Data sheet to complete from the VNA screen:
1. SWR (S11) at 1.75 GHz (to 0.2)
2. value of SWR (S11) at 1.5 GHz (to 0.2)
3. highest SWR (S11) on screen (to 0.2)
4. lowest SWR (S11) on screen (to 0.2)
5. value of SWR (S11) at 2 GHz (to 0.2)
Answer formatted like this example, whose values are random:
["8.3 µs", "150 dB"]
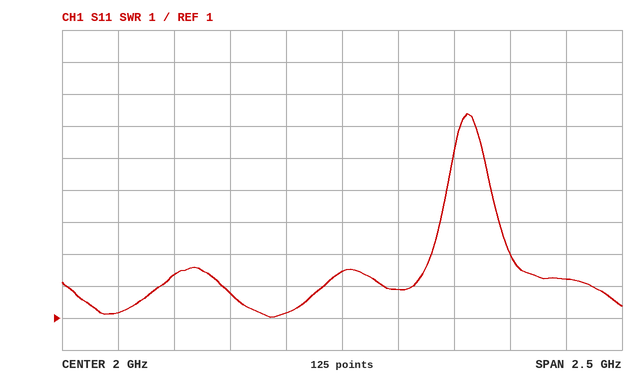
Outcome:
["1.2", "1.8", "7.4", "1.0", "2.4"]
